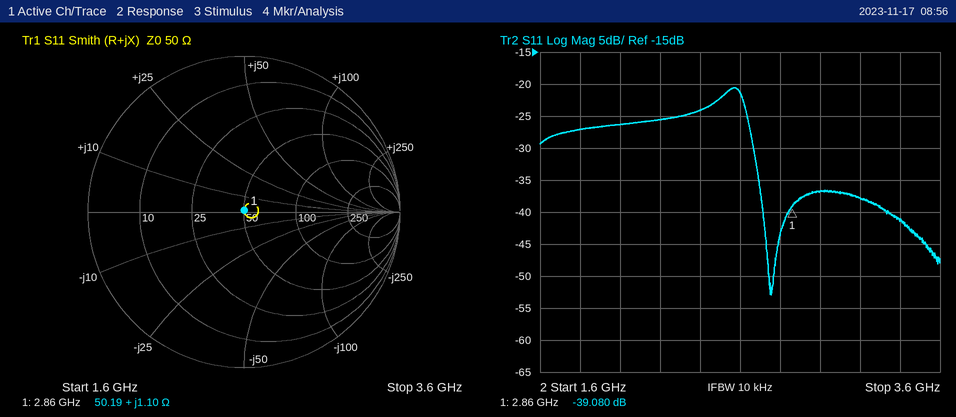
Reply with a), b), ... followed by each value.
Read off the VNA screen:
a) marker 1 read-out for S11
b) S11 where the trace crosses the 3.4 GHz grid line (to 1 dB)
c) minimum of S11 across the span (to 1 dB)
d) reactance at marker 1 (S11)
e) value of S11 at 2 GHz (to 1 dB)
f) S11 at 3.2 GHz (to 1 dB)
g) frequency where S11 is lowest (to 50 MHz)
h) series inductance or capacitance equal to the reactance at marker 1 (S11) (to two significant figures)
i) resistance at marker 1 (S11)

a) -39.080 dB
b) -41 dB
c) -53 dB
d) +1.10 Ω
e) -26 dB
f) -38 dB
g) 2.75 GHz
h) 61 pH
i) 50.19 Ω
